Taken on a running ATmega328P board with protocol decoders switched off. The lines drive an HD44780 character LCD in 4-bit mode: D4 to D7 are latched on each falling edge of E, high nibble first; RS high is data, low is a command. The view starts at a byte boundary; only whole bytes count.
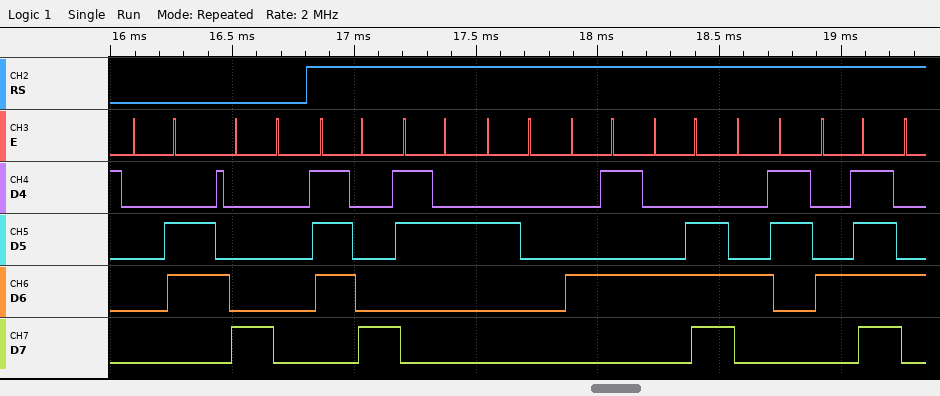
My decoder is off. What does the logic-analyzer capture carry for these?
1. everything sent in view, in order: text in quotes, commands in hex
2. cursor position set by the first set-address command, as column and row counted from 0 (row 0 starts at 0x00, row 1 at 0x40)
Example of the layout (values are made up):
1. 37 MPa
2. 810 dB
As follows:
1. 0x06 0x80 "x2 ENCO"
2. column 0, row 0
